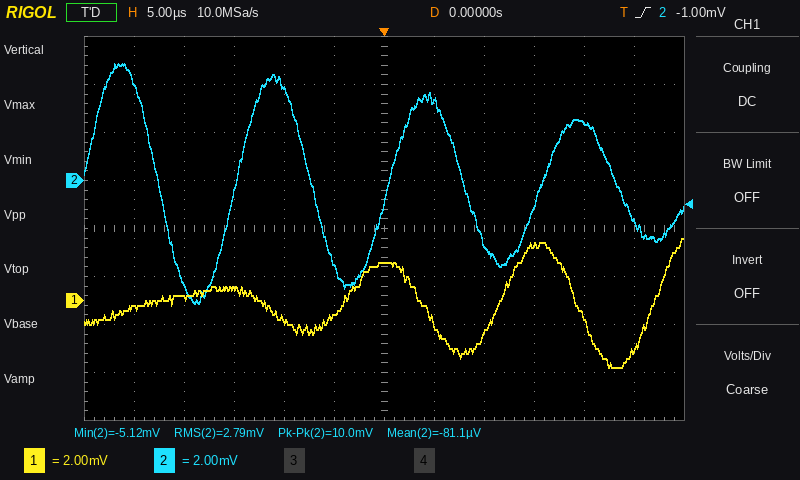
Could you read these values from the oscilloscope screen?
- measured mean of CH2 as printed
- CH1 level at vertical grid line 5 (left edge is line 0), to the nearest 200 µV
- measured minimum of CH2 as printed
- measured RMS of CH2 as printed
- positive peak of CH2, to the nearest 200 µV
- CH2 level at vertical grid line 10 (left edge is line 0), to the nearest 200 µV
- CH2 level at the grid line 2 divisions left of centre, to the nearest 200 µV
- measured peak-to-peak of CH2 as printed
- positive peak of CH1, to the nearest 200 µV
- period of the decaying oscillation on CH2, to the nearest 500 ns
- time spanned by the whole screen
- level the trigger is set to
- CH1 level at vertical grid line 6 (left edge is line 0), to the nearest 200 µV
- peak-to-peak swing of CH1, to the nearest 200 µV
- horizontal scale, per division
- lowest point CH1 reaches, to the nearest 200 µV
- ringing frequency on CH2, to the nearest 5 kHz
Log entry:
-81.1 µV
-600 µV
-5.12 mV
2.79 mV
4.8 mV
2.4 mV
3.8 mV
10.0 mV
2.6 mV
15.0 µs
60 µs
-1.00 mV
1.6 mV
5.4 mV
5 µs
-2.8 mV
65 kHz
